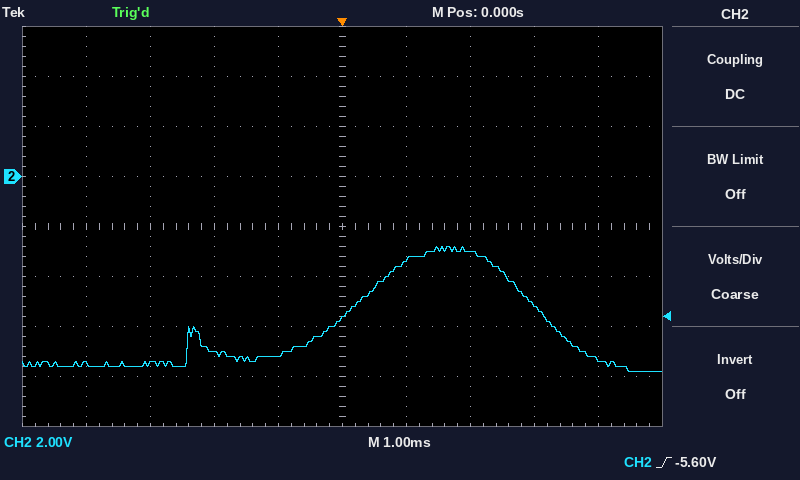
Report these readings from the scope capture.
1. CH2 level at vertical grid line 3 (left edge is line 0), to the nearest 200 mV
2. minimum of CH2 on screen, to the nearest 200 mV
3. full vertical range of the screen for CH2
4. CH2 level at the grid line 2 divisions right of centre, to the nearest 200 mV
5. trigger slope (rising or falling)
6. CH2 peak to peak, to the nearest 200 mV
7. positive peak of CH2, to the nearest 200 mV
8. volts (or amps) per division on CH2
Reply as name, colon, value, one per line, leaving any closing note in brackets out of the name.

CH2 level at vertical grid line 3 (left edge is line 0), to the nearest 200 mV: -7.0 V
minimum of CH2 on screen, to the nearest 200 mV: -7.8 V
full vertical range of the screen for CH2: 16 V
CH2 level at the grid line 2 divisions right of centre, to the nearest 200 mV: -3.0 V
trigger slope: rising
CH2 peak to peak, to the nearest 200 mV: 5.0 V
positive peak of CH2, to the nearest 200 mV: -2.8 V
volts (or amps) per division on CH2: 2 V
